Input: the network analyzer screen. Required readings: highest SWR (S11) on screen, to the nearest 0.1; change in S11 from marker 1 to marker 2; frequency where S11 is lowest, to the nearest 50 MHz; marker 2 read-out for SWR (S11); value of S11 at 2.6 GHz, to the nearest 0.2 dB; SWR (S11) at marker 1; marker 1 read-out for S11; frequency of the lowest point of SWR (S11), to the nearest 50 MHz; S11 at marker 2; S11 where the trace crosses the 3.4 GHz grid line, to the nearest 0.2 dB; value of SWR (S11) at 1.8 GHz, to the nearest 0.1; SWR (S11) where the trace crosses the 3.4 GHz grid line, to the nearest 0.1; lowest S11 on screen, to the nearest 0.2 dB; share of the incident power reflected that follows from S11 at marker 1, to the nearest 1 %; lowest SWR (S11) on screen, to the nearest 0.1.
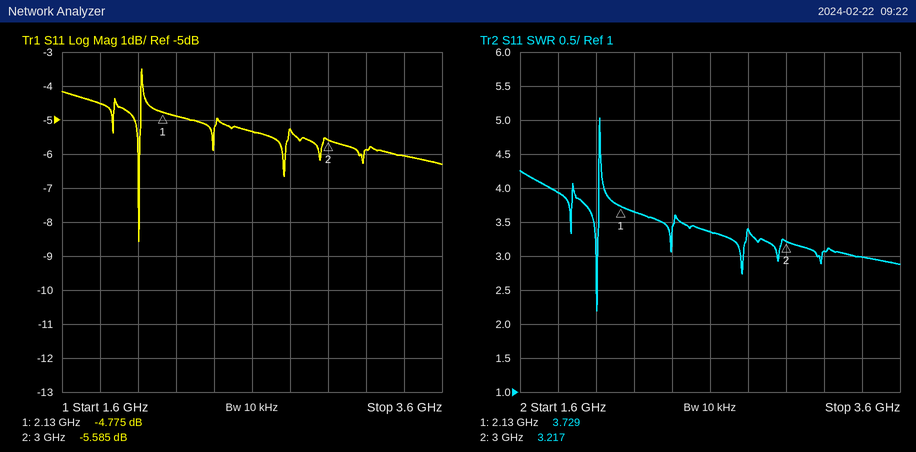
5.0
-0.810 dB
2.00 GHz
3.217
-5.4 dB
3.729
-4.775 dB
2.00 GHz
-5.585 dB
-6.0 dB
3.9
3.0
-8.6 dB
33 %
2.2
